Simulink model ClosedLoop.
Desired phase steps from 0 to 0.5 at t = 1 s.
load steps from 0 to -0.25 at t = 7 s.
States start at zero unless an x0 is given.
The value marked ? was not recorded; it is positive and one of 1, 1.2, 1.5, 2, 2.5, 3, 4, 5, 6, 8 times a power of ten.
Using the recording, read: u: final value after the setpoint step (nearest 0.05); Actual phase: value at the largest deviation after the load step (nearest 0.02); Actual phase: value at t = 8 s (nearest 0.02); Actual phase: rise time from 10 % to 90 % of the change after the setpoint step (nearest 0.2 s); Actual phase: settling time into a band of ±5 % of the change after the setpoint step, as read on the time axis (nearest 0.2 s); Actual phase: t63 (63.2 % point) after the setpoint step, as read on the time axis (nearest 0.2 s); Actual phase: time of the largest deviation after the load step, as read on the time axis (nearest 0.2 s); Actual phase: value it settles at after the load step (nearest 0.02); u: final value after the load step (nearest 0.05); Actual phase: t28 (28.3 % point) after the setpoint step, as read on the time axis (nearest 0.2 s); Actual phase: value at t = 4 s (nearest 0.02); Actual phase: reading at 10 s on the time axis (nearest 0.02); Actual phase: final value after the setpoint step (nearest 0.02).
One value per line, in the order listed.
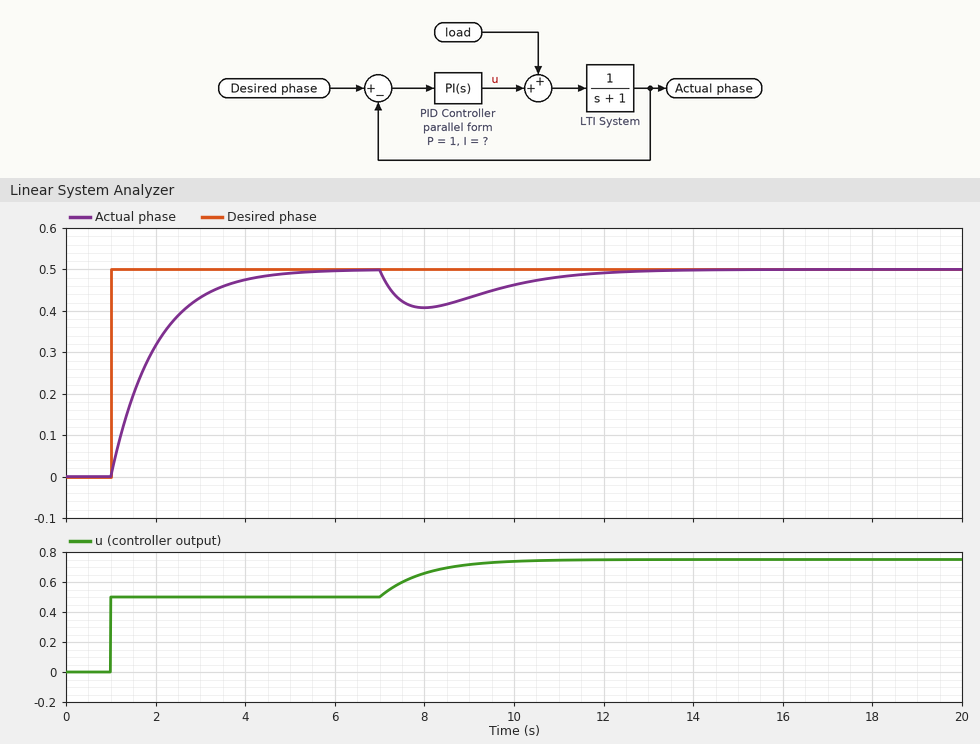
0.50
0.40
0.40
2.2 s
4.0 s
2.0 s
8.0 s
0.50
0.75
1.4 s
0.48
0.46
0.50
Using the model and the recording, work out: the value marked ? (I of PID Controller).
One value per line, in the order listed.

1
